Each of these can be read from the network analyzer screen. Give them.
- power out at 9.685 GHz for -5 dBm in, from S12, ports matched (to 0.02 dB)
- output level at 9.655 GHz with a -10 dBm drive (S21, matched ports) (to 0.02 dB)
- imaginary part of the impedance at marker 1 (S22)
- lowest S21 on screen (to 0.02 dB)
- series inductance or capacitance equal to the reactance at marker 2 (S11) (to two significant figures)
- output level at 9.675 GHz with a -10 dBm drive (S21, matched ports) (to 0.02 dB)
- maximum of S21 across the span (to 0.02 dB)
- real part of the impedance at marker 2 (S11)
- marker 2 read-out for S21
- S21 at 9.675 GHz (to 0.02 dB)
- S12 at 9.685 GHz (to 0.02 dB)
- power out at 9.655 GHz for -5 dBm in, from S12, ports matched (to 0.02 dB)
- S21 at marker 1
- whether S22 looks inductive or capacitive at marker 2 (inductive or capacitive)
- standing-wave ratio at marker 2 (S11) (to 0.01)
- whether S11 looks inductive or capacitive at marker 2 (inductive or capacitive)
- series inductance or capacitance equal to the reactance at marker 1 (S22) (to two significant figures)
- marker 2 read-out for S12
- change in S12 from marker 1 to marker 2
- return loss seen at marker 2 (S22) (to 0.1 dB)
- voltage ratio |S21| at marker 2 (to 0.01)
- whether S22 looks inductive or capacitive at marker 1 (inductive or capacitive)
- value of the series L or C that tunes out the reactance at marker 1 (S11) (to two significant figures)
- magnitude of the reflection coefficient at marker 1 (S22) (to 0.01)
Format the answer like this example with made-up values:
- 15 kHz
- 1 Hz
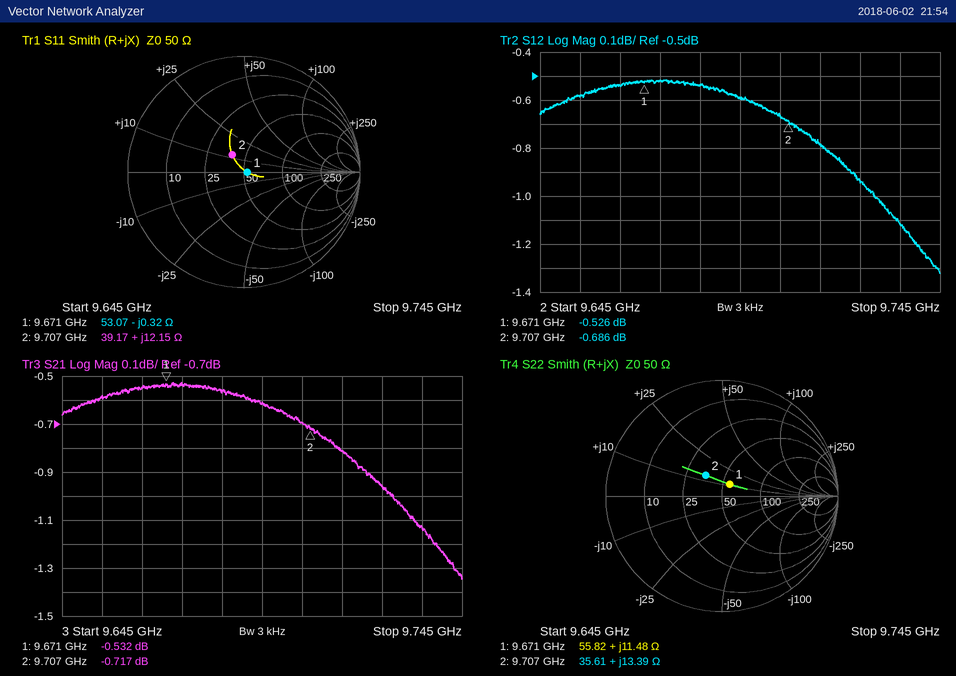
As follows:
- -5.54 dBm
- -10.58 dBm
- +11.48 Ω
- -1.34 dB
- 200 pH
- -10.54 dBm
- -0.52 dB
- 39.17 Ω
- -0.717 dB
- -0.54 dB
- -0.54 dB
- -5.58 dBm
- -0.532 dB
- inductive
- 1.44
- inductive
- 190 pH
- -0.686 dB
- -0.160 dB
- 12.9 dB
- 0.92
- inductive
- 5.3 pH
- 0.12
